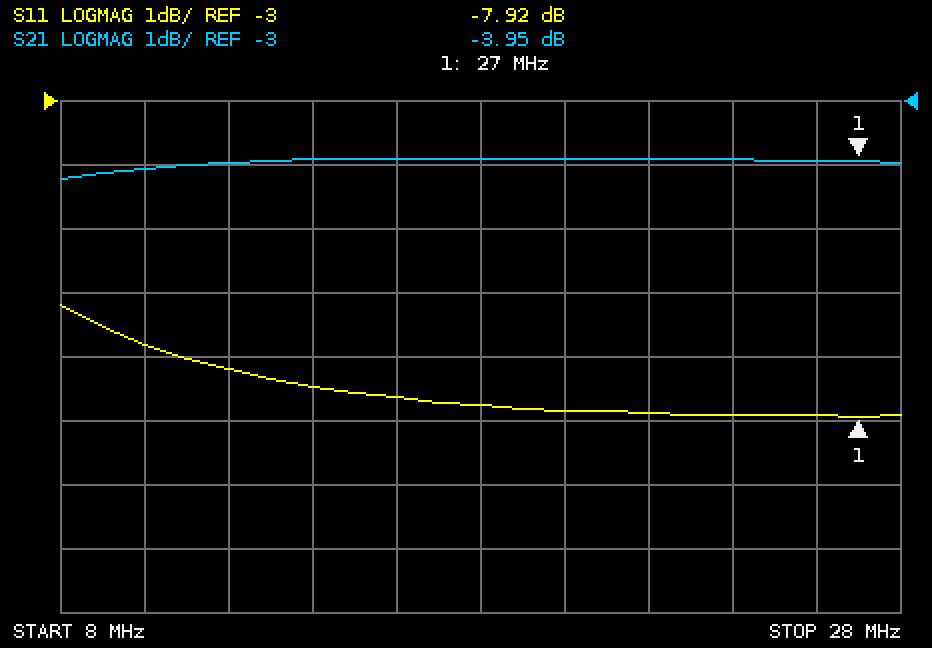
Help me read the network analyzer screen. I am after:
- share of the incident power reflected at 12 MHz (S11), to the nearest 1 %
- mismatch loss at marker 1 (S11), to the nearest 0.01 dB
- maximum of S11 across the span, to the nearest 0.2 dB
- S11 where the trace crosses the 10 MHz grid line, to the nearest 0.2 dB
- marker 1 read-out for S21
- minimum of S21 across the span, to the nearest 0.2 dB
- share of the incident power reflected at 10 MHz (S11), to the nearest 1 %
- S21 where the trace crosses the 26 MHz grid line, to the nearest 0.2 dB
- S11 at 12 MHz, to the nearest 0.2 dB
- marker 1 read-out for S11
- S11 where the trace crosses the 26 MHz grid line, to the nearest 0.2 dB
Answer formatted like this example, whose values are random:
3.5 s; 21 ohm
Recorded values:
19 %; 0.76 dB; -6.2 dB; -6.8 dB; -3.95 dB; -4.2 dB; 21 %; -4.0 dB; -7.2 dB; -7.92 dB; -8.0 dB
